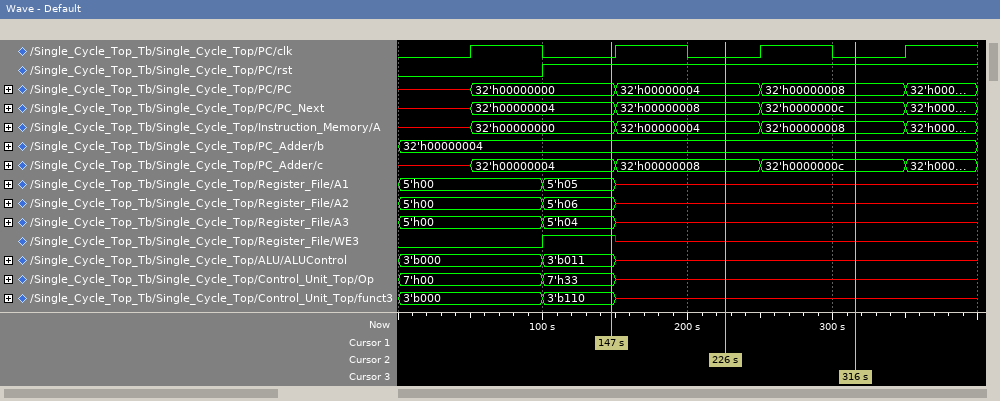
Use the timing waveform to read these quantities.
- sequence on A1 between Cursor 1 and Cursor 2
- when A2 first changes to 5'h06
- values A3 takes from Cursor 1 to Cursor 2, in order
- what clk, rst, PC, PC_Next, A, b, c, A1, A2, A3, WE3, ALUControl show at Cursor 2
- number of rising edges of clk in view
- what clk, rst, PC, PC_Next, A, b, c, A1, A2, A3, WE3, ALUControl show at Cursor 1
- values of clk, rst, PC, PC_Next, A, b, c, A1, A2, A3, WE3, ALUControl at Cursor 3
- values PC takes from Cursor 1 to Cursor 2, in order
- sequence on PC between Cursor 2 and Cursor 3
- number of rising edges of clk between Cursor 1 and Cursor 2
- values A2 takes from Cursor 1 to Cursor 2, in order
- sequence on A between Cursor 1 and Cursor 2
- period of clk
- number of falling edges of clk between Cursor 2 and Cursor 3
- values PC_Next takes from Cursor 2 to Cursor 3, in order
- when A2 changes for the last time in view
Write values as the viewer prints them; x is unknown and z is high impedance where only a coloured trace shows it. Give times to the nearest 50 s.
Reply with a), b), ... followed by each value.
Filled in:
a) 5'h05, x
b) 100 s
c) 5'h04, x
d) clk=0, rst=1, PC=32'h00000004, PC_Next=32'h00000008, A=32'h00000004, b=32'h00000004, c=32'h00000008, A1=x, A2=x, A3=x, WE3=x, ALUControl=x
e) 4
f) clk=0, rst=1, PC=32'h00000000, PC_Next=32'h00000004, A=32'h00000000, b=32'h00000004, c=32'h00000004, A1=5'h05, A2=5'h06, A3=5'h04, WE3=1, ALUControl=3'b011
g) clk=0, rst=1, PC=32'h00000008, PC_Next=32'h0000000c, A=32'h00000008, b=32'h00000004, c=32'h0000000c, A1=x, A2=x, A3=x, WE3=x, ALUControl=x
h) 32'h00000000, 32'h00000004
i) 32'h00000004, 32'h00000008
j) 1
k) 5'h06, x
l) 32'h00000000, 32'h00000004
m) 100 s
n) 1
o) 32'h00000008, 32'h0000000c
p) 150 s
